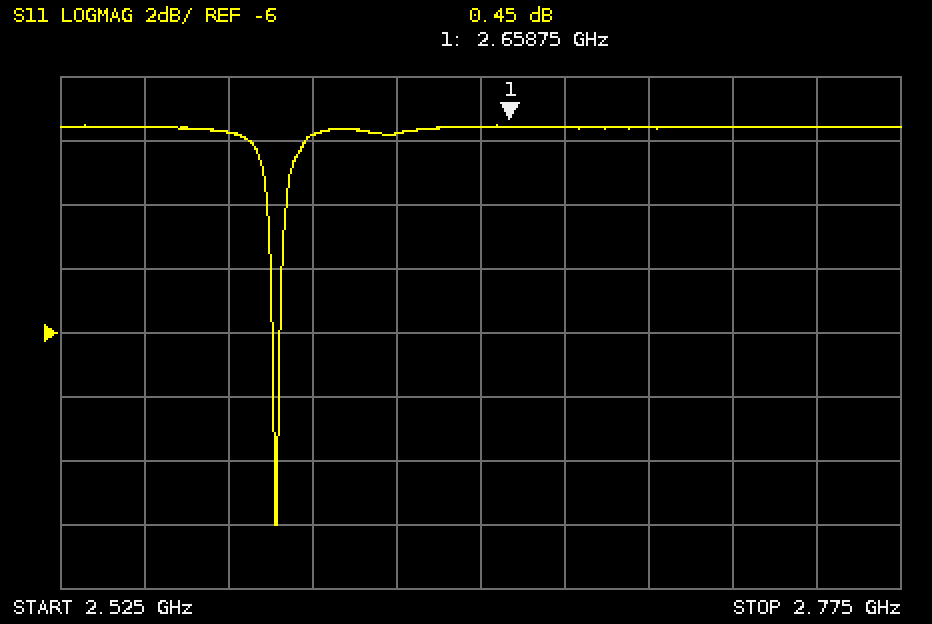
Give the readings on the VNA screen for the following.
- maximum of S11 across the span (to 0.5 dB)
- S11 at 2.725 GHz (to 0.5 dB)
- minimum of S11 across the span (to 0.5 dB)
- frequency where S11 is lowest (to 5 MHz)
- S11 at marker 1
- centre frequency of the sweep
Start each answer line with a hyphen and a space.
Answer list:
- 0.5 dB
- 0.5 dB
- -12.0 dB
- 2.590 GHz
- 0.45 dB
- 2.65 GHz
